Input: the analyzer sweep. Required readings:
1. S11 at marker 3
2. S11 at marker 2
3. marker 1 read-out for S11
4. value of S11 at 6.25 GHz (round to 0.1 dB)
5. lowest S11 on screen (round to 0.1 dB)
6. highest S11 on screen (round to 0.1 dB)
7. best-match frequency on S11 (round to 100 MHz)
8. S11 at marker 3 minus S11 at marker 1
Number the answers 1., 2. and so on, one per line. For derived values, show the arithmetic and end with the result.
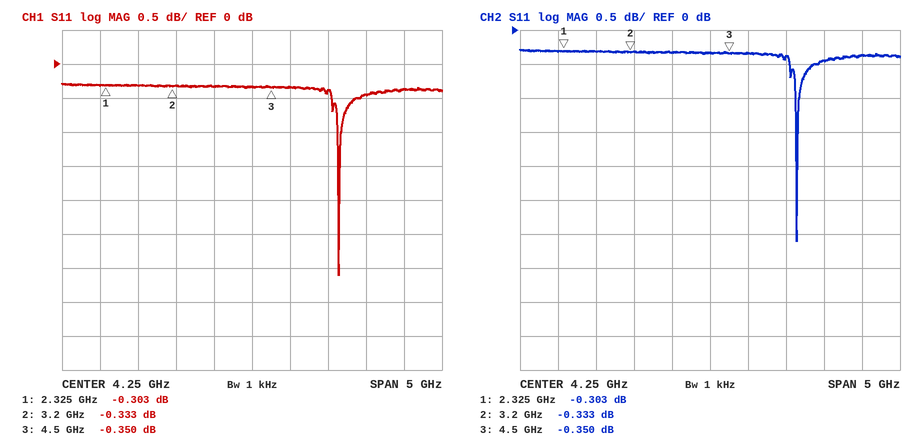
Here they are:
1. -0.350 dB
2. -0.333 dB
3. -0.303 dB
4. -0.4 dB
5. -3.1 dB
6. -0.3 dB
7. 5.4 GHz
8. -0.35 − (-0.303) = -0.047 dB
